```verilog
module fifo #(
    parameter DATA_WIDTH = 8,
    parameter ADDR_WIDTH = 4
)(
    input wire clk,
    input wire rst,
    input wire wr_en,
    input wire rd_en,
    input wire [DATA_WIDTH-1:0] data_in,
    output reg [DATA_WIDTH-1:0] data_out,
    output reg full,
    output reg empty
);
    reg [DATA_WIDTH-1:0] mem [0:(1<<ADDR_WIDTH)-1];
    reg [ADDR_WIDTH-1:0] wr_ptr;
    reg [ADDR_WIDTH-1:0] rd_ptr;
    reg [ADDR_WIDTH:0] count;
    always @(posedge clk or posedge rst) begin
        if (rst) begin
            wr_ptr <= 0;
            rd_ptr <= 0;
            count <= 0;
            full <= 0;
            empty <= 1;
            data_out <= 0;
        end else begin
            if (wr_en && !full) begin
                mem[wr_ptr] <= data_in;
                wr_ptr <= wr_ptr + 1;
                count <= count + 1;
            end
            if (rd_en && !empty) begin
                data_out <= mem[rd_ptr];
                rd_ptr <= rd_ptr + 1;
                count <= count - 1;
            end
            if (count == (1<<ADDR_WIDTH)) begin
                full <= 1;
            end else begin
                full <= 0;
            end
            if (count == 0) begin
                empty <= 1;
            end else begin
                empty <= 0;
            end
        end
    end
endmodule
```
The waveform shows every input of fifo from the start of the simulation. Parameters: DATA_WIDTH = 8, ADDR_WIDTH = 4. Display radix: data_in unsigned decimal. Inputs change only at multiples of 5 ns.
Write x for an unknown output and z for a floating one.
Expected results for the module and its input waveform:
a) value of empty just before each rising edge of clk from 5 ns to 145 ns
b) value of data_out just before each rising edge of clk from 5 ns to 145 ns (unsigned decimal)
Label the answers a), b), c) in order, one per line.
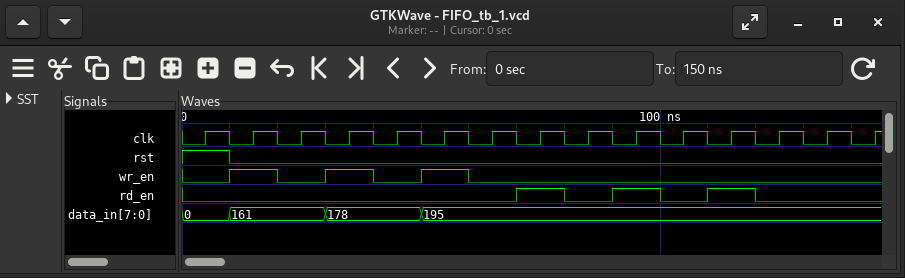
a) 1 1 1 0 0 0 0 0 0 0 0 0 0 1 1
b) 0, 0, 0, 0, 0, 0, 0, 0, 161, 161, 178, 178, 195, 195, 195
